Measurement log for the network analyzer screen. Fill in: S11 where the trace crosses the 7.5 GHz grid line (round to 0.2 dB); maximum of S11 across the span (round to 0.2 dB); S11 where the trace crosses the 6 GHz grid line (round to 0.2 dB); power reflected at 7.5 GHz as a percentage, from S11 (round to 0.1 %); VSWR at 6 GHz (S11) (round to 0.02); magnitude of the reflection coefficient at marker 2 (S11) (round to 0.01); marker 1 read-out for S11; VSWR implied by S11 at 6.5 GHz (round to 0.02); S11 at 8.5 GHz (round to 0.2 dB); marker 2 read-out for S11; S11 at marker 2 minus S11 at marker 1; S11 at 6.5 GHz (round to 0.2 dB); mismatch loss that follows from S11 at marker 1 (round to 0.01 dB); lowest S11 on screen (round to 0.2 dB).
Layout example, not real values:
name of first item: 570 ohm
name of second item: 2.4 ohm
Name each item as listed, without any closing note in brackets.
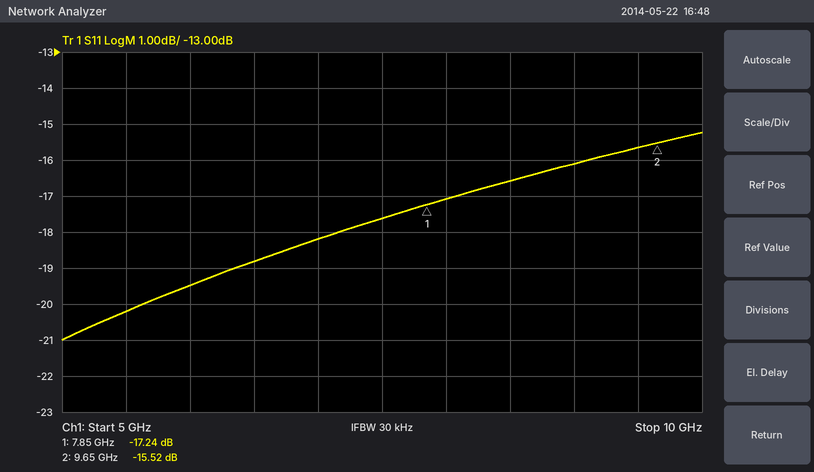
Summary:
S11 where the trace crosses the 7.5 GHz grid line: -17.6 dB
maximum of S11 across the span: -15.2 dB
S11 where the trace crosses the 6 GHz grid line: -19.4 dB
power reflected at 7.5 GHz as a percentage, from S11: 1.7 %
VSWR at 6 GHz (S11): 1.24
magnitude of the reflection coefficient at marker 2 (S11): 0.17
marker 1 read-out for S11: -17.24 dB
VSWR implied by S11 at 6.5 GHz: 1.26
S11 at 8.5 GHz: -16.6 dB
marker 2 read-out for S11: -15.52 dB
S11 at marker 2 minus S11 at marker 1: 1.72 dB
S11 at 6.5 GHz: -18.8 dB
mismatch loss that follows from S11 at marker 1: 0.08 dB
lowest S11 on screen: -21.0 dB
